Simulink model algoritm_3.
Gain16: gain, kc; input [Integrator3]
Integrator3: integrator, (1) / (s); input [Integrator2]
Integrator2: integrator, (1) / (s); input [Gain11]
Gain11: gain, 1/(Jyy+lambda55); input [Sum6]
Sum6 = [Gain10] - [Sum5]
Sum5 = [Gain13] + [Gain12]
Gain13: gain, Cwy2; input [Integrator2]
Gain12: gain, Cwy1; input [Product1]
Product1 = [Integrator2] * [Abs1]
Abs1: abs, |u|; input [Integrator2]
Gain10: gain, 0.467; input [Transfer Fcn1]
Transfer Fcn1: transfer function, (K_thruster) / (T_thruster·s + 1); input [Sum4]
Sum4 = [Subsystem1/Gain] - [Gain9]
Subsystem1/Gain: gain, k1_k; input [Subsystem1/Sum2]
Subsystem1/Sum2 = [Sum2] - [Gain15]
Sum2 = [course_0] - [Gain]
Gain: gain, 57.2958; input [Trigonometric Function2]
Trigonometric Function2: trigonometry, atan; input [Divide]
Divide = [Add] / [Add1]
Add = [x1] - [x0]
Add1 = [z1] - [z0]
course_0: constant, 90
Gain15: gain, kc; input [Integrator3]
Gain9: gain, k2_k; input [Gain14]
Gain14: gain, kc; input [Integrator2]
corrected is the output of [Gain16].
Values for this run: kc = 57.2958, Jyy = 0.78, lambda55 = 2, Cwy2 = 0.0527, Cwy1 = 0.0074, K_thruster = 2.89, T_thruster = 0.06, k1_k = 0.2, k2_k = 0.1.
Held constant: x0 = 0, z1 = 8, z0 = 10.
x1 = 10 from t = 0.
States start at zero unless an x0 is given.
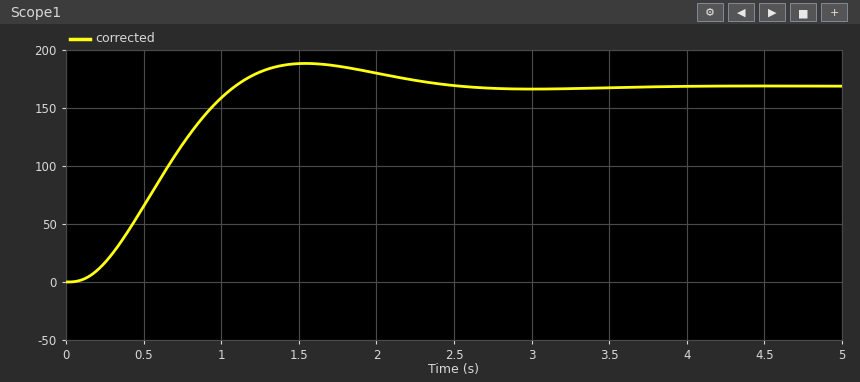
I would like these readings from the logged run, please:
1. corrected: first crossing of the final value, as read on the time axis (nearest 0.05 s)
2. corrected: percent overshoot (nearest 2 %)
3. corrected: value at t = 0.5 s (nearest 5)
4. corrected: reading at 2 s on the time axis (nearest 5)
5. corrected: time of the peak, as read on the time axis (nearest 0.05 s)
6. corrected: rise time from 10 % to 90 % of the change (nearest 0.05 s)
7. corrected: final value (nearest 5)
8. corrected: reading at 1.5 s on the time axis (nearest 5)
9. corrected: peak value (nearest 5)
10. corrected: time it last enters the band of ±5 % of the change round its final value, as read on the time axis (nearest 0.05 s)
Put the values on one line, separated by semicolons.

1.10 s; 12 %; 65; 180; 1.55 s; 0.70 s; 170; 190; 190; 2.10 s
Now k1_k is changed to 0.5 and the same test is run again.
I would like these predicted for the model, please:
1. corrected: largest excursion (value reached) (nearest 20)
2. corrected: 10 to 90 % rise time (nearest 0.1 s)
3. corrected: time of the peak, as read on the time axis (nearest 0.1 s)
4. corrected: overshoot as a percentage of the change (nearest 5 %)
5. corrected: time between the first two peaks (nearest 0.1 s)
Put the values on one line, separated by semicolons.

240; 0.3 s; 0.9 s; 40 %; 1.6 s
